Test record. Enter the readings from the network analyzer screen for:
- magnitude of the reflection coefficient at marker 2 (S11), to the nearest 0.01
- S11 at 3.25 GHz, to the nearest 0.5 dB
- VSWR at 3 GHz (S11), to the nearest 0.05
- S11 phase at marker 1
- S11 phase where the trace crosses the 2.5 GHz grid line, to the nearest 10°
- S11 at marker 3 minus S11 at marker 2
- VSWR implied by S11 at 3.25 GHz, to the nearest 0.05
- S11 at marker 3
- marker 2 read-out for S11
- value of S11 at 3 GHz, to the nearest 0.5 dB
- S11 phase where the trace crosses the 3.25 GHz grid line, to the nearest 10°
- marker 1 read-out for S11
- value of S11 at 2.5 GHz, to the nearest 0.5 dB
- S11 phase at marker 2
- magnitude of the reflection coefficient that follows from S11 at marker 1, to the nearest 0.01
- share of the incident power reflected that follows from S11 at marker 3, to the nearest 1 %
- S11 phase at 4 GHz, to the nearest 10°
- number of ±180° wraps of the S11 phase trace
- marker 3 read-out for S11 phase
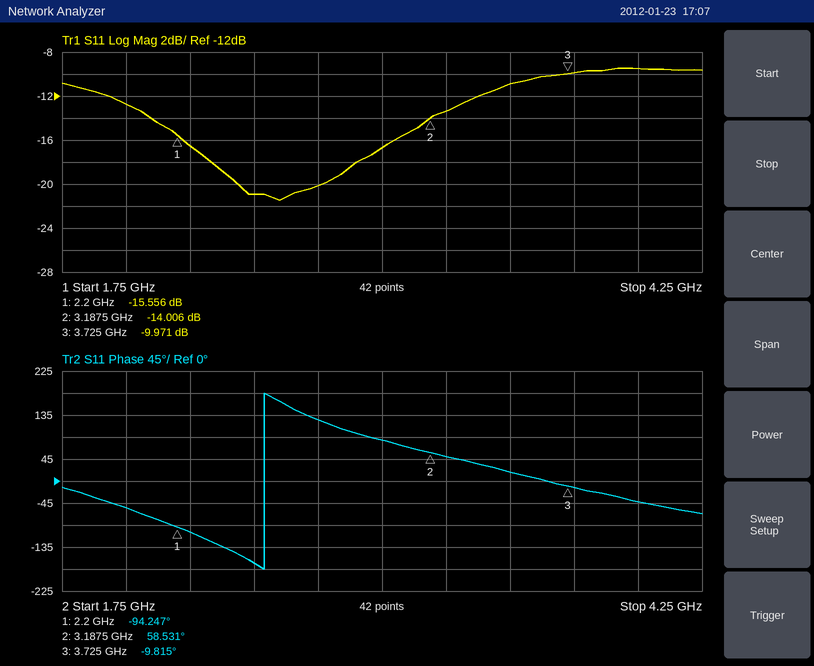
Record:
0.20
-13.5 dB
1.35
-94.247°
-170°
4.035 dB
1.55
-9.971 dB
-14.006 dB
-16.5 dB
50°
-15.556 dB
-21.0 dB
58.531°
0.17
10 %
-40°
1
-9.815°
